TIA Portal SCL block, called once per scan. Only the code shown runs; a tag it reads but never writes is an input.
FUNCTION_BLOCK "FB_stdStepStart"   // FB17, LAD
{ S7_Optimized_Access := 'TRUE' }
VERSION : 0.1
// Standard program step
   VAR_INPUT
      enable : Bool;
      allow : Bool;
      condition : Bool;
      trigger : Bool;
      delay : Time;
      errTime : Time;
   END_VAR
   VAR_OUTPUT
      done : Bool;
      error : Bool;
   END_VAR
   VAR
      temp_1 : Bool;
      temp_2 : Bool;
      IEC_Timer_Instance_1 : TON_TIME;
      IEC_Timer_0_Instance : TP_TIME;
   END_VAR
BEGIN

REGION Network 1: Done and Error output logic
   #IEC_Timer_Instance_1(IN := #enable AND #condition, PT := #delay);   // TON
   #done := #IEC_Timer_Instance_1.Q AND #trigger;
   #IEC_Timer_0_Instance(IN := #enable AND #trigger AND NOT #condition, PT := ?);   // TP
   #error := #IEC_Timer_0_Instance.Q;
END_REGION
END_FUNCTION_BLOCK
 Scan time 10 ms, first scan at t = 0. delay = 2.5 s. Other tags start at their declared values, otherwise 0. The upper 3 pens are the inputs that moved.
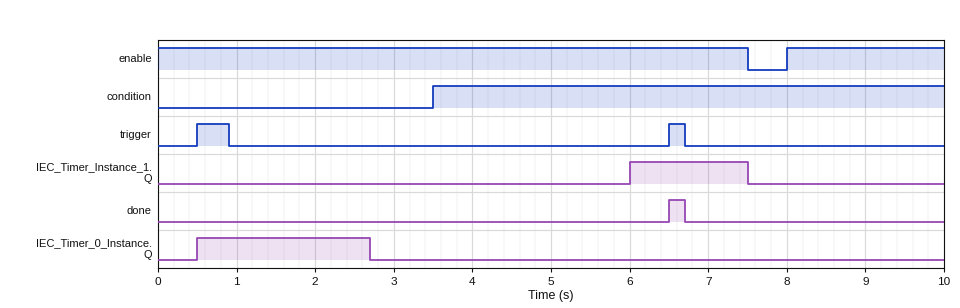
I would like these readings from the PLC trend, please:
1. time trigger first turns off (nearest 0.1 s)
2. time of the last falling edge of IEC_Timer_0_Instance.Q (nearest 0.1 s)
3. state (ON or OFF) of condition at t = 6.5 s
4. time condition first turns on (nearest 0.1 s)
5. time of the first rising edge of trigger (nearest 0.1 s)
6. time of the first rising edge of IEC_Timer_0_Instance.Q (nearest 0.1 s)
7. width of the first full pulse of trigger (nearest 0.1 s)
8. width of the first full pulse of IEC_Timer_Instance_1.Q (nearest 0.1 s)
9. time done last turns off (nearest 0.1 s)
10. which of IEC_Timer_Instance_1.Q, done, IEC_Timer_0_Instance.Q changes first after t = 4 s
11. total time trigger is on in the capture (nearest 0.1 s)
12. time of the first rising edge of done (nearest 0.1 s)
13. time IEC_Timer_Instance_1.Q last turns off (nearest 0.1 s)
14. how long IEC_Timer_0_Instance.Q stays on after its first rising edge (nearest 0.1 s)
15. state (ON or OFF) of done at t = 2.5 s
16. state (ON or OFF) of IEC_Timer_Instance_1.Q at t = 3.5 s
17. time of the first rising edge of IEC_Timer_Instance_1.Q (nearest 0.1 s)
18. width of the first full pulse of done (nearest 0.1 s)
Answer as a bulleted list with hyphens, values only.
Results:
- 0.9 s
- 2.7 s
- ON
- 3.5 s
- 0.5 s
- 0.5 s
- 0.4 s
- 1.5 s
- 6.7 s
- IEC_Timer_Instance_1.Q
- 0.6 s
- 6.5 s
- 7.5 s
- 2.2 s
- OFF
- OFF
- 6.0 s
- 0.2 s
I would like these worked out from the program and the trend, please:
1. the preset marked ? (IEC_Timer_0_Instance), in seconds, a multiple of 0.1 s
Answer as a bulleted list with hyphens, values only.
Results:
- 2.2 s
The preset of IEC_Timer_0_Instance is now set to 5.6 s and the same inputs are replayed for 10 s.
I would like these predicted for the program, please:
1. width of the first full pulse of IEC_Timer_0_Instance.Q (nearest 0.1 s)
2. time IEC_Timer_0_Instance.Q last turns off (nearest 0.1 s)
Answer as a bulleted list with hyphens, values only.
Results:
- 5.6 s
- 6.1 s
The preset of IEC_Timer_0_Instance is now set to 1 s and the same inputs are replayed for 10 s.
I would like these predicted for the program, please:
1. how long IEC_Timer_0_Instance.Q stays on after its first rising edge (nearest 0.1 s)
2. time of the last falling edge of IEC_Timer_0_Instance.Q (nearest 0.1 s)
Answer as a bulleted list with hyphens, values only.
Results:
- 1.0 s
- 1.5 s
